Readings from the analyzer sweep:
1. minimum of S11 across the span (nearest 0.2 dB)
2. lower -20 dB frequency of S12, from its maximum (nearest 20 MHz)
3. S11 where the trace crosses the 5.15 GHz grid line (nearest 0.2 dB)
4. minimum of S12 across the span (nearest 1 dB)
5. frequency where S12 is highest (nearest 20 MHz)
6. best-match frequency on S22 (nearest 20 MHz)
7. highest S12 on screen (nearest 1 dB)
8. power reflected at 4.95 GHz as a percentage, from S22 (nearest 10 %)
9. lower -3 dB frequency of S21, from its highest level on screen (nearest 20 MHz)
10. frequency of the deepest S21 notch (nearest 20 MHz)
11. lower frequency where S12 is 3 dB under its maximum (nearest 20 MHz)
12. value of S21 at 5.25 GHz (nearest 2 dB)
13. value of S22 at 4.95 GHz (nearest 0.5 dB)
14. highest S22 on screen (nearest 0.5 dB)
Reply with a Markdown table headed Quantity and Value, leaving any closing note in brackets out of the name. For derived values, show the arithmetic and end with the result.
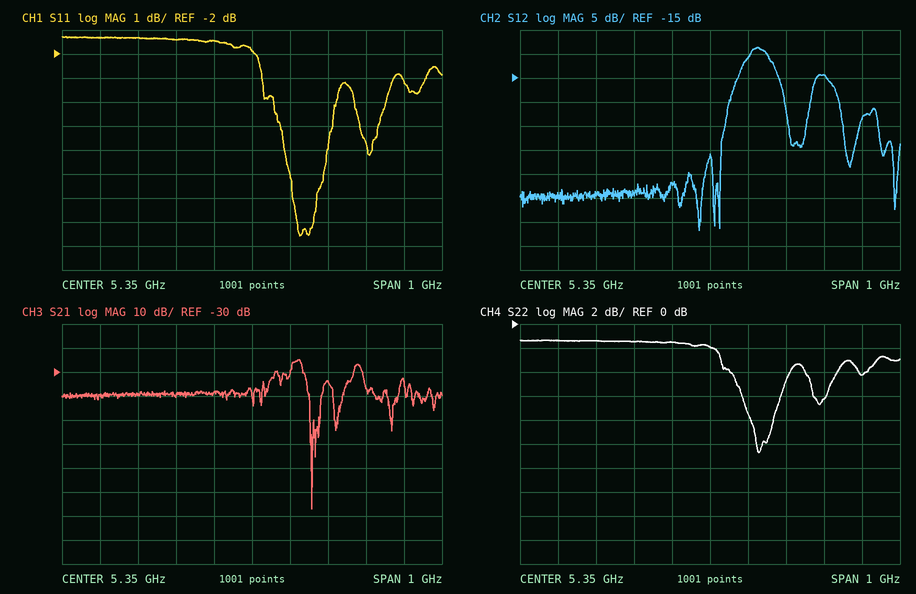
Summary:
| Quantity | Value |
|---|---|
| minimum of S11 across the span | -9.6 dB |
| lower -20 dB frequency of S12, from its maximum | 5.38 GHz |
| S11 where the trace crosses the 5.15 GHz grid line | -1.4 dB |
| minimum of S12 across the span | -47 dB |
| frequency where S12 is highest | 5.48 GHz |
| best-match frequency on S22 | 5.48 GHz |
| highest S12 on screen | -9 dB |
| power reflected at 4.95 GHz as a percentage, from S22 | 10^(-1.5/10) ≈ 70.8 %, so 70 % to the nearest 10 % |
| lower -3 dB frequency of S21, from its highest level on screen | 5.46 GHz |
| frequency of the deepest S21 notch | 5.50 GHz |
| lower frequency where S12 is 3 dB under its maximum | 5.44 GHz |
| value of S21 at 5.25 GHz | -38 dB |
| value of S22 at 4.95 GHz | -1.5 dB |
| highest S22 on screen | -1.5 dB |
